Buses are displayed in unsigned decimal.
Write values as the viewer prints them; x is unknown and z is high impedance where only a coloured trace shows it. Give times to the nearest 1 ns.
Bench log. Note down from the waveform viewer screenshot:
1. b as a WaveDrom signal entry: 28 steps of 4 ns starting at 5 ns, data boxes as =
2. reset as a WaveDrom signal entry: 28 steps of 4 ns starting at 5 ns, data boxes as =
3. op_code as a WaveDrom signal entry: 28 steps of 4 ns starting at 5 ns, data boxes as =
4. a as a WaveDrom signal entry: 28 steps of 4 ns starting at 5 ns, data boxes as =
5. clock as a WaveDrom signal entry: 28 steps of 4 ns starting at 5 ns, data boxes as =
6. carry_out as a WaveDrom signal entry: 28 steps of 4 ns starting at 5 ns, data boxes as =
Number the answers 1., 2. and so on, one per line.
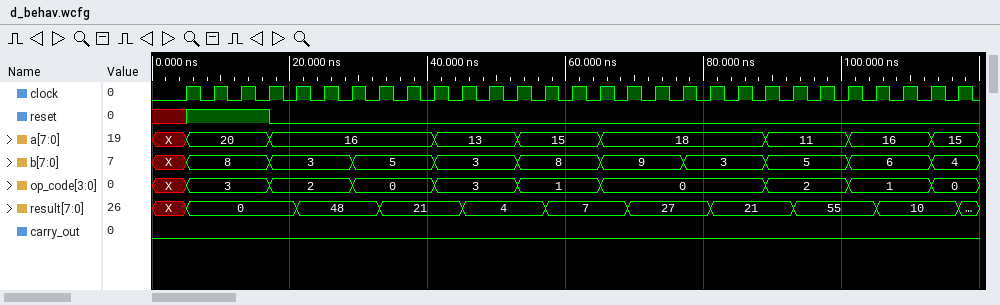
1. {name: 'b', wave: '=..=..=..=..=..=..=..=..=..=', data: '8 3 5 3 8 9 3 5 6 4'}
2. {name: 'reset', wave: '1..0........................'}
3. {name: 'op_code', wave: '=..=..=..=..=..=.....=..=..=', data: '3 2 0 3 1 0 2 1 0'}
4. {name: 'a', wave: '=..=.....=..=..=.....=..=..=', data: '20 16 13 15 18 11 16 15'}
5. {name: 'clock', wave: 'p...........................'}
6. {name: 'carry_out', wave: '0...........................'}
